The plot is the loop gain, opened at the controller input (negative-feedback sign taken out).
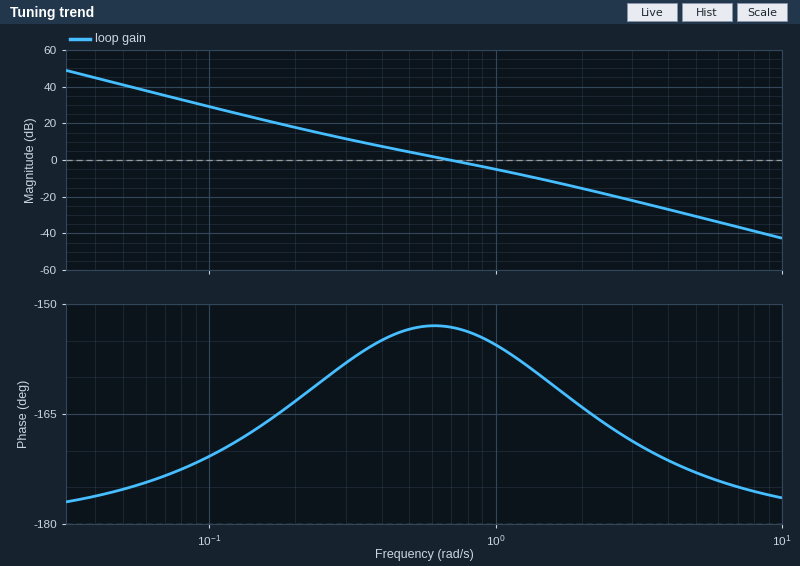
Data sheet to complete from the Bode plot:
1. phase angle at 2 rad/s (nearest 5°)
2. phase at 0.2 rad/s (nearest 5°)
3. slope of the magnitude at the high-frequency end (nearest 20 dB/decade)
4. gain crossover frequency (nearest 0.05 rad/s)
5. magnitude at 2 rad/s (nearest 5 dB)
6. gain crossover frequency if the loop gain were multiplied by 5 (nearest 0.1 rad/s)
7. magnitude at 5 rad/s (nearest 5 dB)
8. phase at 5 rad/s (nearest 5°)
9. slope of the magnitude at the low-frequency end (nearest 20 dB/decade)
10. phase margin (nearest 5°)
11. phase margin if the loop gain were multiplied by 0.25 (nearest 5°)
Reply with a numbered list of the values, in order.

1. -165°
2. -165°
3. -40 dB/decade
4. 0.70 rad/s
5. -15 dB
6. 1.8 rad/s
7. -30 dB
8. -175°
9. -40 dB/decade
10. 25°
11. 20°
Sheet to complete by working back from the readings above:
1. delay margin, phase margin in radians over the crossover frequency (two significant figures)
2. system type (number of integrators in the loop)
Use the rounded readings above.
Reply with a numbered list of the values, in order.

1. 0.62 s
2. 2
